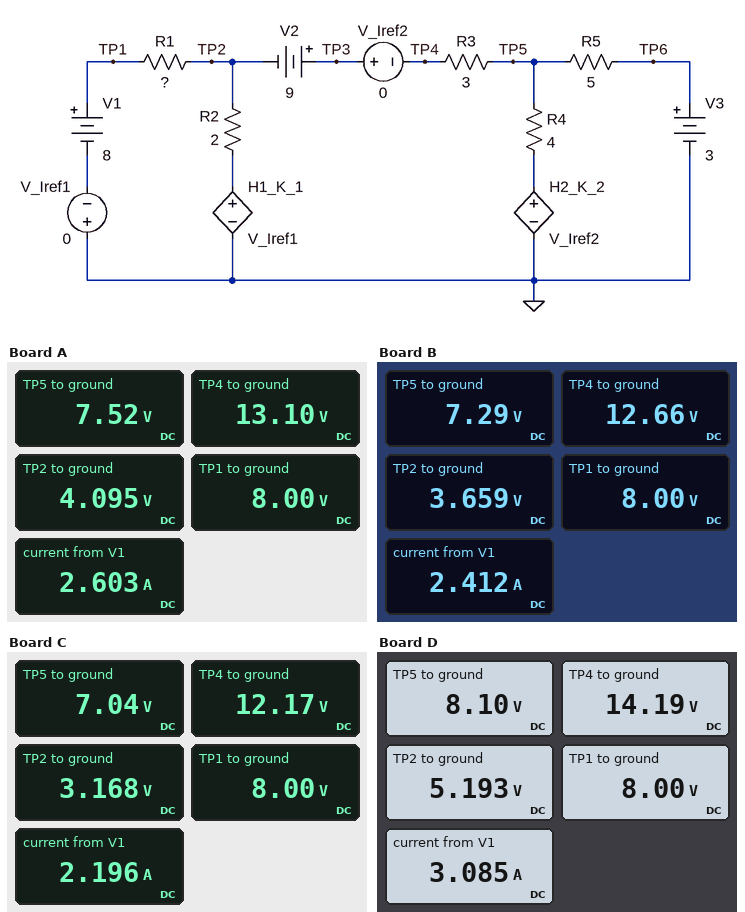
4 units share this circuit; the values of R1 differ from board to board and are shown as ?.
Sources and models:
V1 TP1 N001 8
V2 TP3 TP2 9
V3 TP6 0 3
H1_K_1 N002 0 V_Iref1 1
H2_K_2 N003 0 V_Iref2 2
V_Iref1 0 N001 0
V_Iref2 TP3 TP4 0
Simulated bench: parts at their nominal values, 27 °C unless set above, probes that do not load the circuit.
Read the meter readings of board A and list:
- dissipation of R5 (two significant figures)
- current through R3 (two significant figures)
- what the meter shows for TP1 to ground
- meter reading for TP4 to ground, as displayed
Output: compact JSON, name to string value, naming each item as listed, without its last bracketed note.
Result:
{"dissipation of R5": "4.1 W", "current through R3": "1.9 A", "what the meter shows for TP1 to ground": "8.00 V", "meter reading for TP4 to ground, as displayed": "13.10 V"}
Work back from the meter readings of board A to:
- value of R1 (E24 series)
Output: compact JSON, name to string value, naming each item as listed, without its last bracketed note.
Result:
{"value of R1": "1.5 Ω"}
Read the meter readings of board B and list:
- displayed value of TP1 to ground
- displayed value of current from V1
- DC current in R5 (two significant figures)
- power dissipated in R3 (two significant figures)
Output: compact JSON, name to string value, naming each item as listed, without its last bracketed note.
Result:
{"displayed value of TP1 to ground": "8.00 V", "displayed value of current from V1": "2.412 A", "DC current in R5": "860 mA", "power dissipated in R3": "9.6 W"}
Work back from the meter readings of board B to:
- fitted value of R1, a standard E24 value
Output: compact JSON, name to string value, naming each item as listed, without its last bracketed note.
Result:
{"fitted value of R1, a standard E24 value": "1.8 Ω"}
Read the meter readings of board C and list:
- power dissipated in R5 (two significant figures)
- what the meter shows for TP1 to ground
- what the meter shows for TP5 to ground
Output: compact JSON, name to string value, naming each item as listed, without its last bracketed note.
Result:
{"power dissipated in R5": "3.3 W", "what the meter shows for TP1 to ground": "8.00 V", "what the meter shows for TP5 to ground": "7.04 V"}
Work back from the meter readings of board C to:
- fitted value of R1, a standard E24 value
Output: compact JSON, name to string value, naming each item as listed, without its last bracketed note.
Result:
{"fitted value of R1, a standard E24 value": "2.2 Ω"}
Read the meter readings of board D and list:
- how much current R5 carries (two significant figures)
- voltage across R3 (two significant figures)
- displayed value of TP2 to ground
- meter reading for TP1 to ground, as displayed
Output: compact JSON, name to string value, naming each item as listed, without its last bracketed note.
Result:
{"how much current R5 carries": "1.0 A", "voltage across R3": "6.1 V", "displayed value of TP2 to ground": "5.193 V", "meter reading for TP1 to ground, as displayed": "8.00 V"}
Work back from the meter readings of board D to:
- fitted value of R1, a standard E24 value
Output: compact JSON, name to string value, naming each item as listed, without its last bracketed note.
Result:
{"fitted value of R1, a standard E24 value": "0.91 Ω"}
